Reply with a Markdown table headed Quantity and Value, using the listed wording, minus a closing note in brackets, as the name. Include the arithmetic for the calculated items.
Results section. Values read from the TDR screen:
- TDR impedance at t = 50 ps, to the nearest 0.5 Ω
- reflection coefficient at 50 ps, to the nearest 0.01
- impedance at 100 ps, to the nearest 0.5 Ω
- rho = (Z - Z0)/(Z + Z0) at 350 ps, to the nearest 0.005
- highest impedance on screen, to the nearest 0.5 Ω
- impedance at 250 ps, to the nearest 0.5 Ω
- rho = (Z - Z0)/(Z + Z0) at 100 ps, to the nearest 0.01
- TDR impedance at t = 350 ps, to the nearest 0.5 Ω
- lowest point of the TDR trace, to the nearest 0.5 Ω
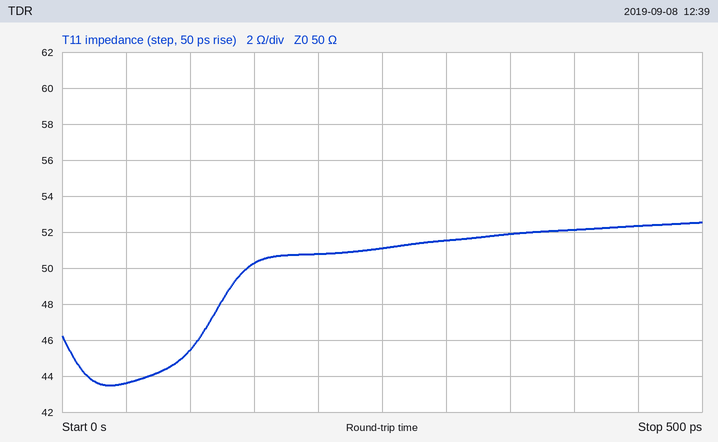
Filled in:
| Quantity | Value |
|---|---|
| TDR impedance at t = 50 ps, to the nearest 0.5 Ω | 43.5 Ω |
| reflection coefficient at 50 ps, to the nearest 0.01 | (43.5 − 50)/(43.5 + 50) ≈ -0.07 |
| impedance at 100 ps, to the nearest 0.5 Ω | 45.5 Ω |
| rho = (Z - Z0)/(Z + Z0) at 350 ps, to the nearest 0.005 | (52 − 50)/(52 + 50) ≈ +0.020 |
| highest impedance on screen, to the nearest 0.5 Ω | 52.5 Ω |
| impedance at 250 ps, to the nearest 0.5 Ω | 51.0 Ω |
| rho = (Z - Z0)/(Z + Z0) at 100 ps, to the nearest 0.01 | (45.5 − 50)/(45.5 + 50) ≈ -0.05 |
| TDR impedance at t = 350 ps, to the nearest 0.5 Ω | 52.0 Ω |
| lowest point of the TDR trace, to the nearest 0.5 Ω | 43.5 Ω |
